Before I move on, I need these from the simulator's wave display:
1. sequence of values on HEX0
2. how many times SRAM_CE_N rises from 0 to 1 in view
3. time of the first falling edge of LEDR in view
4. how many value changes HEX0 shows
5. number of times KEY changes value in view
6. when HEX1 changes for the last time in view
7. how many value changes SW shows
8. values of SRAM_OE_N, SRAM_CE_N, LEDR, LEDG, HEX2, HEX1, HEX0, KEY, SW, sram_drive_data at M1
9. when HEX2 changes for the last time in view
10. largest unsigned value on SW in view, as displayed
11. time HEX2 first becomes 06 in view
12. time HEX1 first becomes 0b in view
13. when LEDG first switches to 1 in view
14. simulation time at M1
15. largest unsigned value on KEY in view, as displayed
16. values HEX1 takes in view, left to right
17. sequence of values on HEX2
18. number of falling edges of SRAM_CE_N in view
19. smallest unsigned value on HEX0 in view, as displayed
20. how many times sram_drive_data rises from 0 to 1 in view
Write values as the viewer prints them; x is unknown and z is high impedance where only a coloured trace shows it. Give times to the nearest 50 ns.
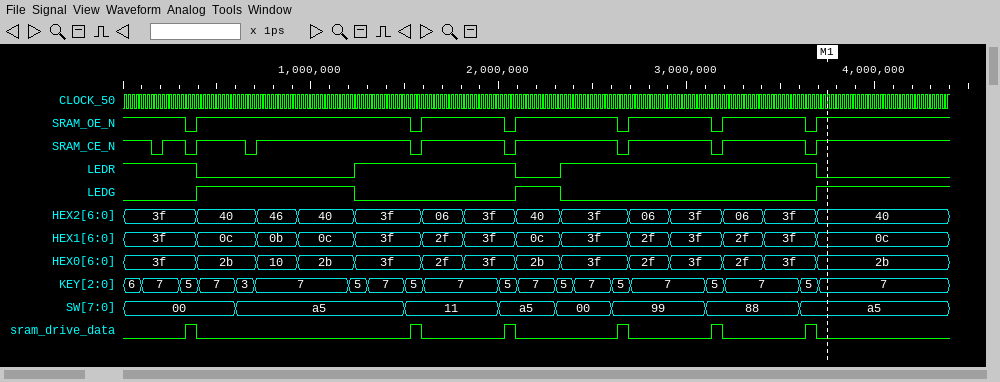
3f, 2b, 10, 2b, 3f, 2f, 3f, 2b, 3f, 2f, 3f, 2f, 3f, 2b
8
400 ns
13
19
3700 ns
7
SRAM_OE_N=1, SRAM_CE_N=1, LEDR=0, LEDG=1, HEX2=40, HEX1=0c, HEX0=2b, KEY=7, SW=a5, sram_drive_data=0
3700 ns
a5
1600 ns
700 ns
400 ns
3750 ns
7
3f, 0c, 0b, 0c, 3f, 2f, 3f, 0c, 3f, 2f, 3f, 2f, 3f, 0c
3f, 40, 46, 40, 3f, 06, 3f, 40, 3f, 06, 3f, 06, 3f, 40
8
10
6
